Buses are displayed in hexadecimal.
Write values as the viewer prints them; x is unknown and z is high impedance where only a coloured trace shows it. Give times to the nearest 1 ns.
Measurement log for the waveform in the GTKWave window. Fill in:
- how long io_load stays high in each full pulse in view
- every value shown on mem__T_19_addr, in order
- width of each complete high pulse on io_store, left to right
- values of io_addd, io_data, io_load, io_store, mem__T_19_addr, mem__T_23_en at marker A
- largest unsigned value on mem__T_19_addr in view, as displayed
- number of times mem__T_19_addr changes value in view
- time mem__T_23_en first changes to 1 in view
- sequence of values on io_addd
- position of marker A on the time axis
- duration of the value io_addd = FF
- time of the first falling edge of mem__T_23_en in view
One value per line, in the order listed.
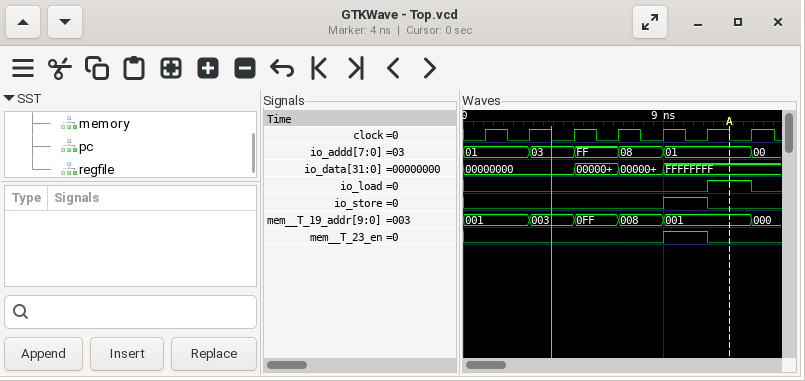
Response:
2 ns
001, 003, 0FF, 008, 001, 000
2 ns
io_addd=01, io_data=FFFFFFFF, io_load=1, io_store=0, mem__T_19_addr=001, mem__T_23_en=0
0FF
5
9 ns
01, 03, FF, 08, 01, 00
12 ns
2 ns
11 ns
